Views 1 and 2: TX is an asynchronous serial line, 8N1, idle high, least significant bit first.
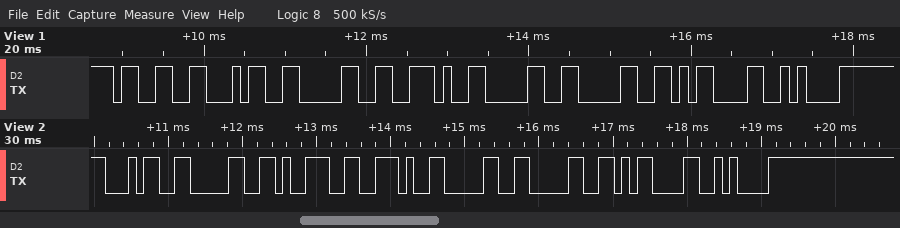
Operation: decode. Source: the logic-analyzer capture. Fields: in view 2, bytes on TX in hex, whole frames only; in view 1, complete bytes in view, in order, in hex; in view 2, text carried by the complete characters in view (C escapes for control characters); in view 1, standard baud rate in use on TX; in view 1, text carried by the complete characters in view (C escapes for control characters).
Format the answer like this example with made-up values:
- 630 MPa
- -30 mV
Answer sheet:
- 34 30 39 2E 30 30 0D 0A
- 33 34 30 2E 30 30 0D 0A
- "409.00\r\n"
- 9600 baud
- "340.00\r\n"
